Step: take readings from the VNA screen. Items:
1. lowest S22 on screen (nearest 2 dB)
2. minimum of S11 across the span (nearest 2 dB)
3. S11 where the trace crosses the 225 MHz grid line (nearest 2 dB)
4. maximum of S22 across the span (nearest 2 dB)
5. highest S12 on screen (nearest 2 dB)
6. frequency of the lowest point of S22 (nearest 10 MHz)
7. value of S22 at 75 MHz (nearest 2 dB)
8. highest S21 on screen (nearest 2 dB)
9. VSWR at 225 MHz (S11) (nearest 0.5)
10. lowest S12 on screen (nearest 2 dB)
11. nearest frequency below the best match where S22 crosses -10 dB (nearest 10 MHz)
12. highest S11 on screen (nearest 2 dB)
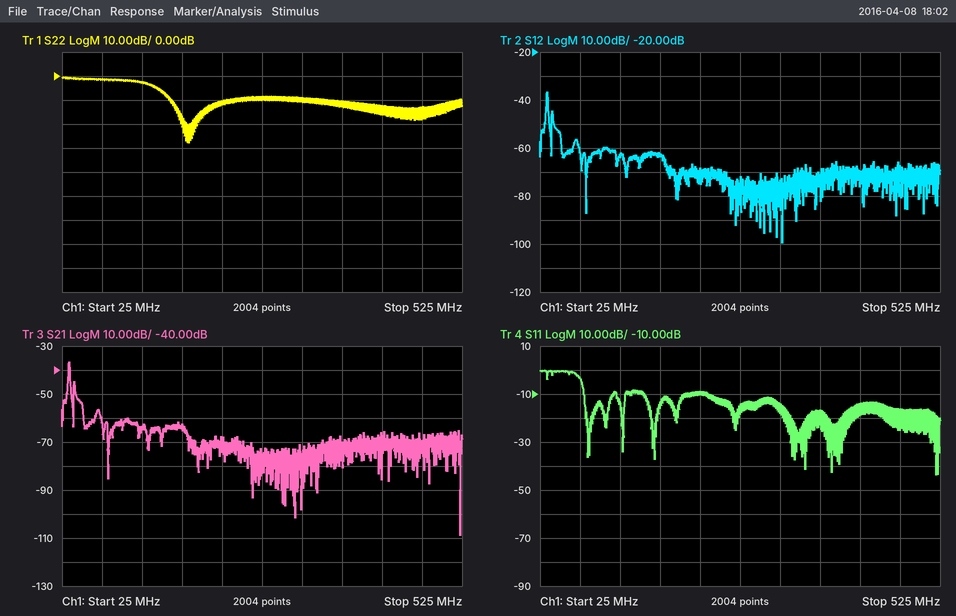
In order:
-28 dB
-44 dB
-10 dB
0 dB
-36 dB
180 MHz
-2 dB
-36 dB
2.0
-100 dB
160 MHz
0 dB
